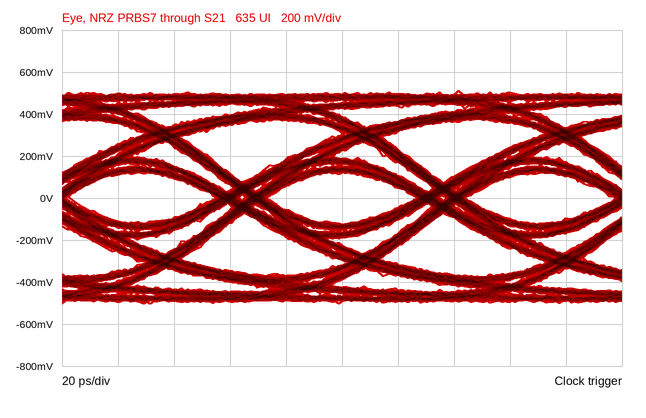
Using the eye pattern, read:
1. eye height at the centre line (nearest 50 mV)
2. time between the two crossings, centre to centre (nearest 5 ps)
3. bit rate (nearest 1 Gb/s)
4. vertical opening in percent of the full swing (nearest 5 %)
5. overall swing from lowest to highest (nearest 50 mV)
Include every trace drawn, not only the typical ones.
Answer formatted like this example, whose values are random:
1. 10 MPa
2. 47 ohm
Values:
1. 250 mV
2. 70 ps
3. 14 Gb/s
4. 25 %
5. 1.00 V
